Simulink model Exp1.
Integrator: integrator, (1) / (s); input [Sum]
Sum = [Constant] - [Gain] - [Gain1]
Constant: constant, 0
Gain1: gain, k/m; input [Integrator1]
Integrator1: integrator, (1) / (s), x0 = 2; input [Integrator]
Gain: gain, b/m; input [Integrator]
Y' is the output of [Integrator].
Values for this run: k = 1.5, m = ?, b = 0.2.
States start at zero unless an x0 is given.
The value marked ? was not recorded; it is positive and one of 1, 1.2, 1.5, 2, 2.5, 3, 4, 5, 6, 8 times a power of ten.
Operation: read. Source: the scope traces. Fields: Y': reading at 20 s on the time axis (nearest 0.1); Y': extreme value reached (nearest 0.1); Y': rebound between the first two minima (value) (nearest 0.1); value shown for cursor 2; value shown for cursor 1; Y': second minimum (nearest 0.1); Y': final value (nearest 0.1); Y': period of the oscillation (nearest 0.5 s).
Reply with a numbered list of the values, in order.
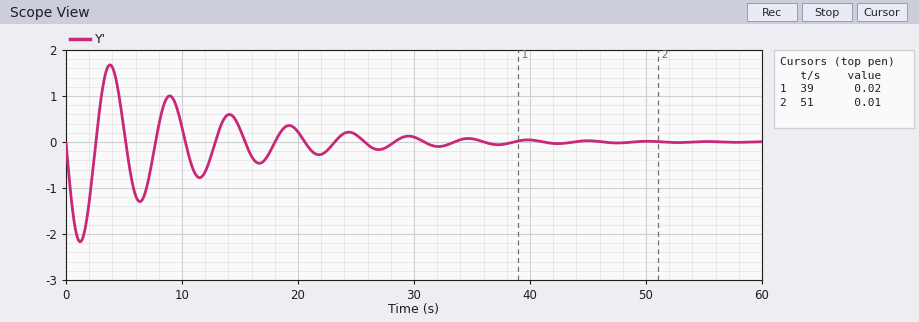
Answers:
1. 0.2
2. -2.2
3. 1.7
4. 0.01
5. 0.02
6. -1.3
7. 0.0
8. 5.0 s
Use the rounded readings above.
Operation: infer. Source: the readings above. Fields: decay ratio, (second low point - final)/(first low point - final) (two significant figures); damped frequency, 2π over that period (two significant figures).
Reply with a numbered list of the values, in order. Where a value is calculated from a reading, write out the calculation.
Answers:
1. (-1.3 - 0) / (-2.2 - 0) = 0.59
2. 2π / 5 = 1.3 rad/s
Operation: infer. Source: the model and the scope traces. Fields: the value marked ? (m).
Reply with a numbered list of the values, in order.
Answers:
1. 1
